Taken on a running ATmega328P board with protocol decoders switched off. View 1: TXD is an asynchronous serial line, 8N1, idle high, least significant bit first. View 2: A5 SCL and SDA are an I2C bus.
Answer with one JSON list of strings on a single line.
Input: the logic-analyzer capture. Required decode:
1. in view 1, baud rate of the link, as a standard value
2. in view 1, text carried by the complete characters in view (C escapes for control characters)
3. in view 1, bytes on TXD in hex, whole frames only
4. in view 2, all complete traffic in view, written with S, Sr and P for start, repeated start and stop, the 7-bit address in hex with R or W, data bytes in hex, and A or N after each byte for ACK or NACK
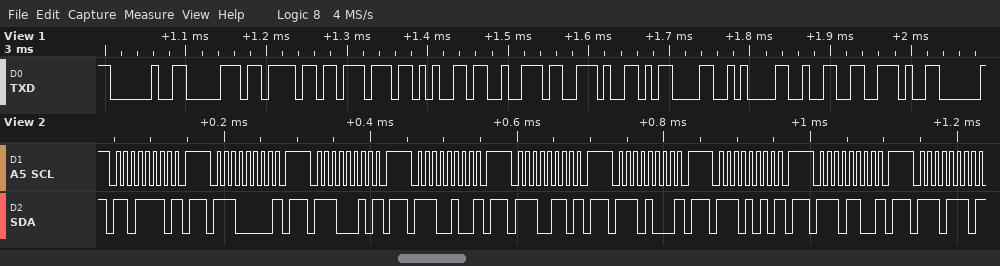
["115200 baud", "\" power.\\r\\n2.\"", "20 70 6F 77 65 72 2E 0D 0A 32 2E", "S 6FW N P S 70W N P S 71W N P S 72W N P S 73W N P S 74W N P S 75W N P S 76W N P S 77W N"]
